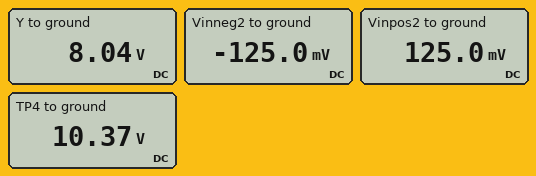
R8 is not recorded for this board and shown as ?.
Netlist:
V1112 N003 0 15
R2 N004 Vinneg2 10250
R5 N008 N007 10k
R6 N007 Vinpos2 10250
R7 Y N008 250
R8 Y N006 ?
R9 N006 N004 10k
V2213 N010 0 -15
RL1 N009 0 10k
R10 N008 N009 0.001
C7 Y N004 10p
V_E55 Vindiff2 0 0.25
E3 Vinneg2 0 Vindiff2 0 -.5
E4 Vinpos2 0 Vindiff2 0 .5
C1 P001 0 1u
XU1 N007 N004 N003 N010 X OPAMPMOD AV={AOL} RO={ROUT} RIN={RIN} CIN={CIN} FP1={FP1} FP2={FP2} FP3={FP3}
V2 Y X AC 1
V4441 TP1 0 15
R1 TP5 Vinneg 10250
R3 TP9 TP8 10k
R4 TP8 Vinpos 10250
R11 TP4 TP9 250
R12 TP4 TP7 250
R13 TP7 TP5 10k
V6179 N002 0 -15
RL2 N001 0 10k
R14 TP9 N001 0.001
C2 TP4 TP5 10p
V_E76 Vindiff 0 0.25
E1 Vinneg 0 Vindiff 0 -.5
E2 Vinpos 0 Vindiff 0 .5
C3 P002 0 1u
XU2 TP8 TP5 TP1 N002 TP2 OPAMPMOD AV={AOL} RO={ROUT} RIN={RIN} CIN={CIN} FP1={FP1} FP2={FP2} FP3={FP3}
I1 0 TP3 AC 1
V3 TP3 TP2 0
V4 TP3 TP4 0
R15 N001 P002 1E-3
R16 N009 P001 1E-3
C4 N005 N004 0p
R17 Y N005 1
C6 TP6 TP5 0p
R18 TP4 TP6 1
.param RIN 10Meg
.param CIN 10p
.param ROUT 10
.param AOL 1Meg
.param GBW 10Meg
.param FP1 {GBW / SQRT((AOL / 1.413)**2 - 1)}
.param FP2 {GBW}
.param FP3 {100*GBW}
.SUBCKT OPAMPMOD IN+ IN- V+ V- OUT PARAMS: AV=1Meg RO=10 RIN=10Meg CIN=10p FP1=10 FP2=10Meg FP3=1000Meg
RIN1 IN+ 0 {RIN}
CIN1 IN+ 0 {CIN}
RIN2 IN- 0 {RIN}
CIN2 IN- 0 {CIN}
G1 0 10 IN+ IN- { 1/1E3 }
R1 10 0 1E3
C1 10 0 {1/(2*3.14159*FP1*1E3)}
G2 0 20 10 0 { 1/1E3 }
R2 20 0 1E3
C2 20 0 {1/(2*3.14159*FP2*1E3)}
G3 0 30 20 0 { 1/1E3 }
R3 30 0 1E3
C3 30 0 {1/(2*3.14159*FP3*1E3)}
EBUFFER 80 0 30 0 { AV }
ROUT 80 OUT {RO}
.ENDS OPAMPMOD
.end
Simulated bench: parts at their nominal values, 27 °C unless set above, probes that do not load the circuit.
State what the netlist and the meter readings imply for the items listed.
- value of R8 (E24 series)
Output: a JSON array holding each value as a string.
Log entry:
["110 Ω"]
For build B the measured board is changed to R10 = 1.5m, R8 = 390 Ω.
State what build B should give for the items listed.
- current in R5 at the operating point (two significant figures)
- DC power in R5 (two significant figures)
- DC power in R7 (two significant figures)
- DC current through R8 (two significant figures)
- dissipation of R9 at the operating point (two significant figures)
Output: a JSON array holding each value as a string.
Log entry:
["680 µA", "4.7 mW", "1.1 mW", "710 µA", "5.0 mW"]
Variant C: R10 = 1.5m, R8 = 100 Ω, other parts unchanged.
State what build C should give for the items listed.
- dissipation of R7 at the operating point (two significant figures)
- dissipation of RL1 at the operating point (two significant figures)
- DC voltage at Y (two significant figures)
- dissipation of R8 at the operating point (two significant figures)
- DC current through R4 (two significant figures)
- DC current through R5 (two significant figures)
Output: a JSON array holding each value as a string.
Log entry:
["320 µW", "5.8 mW", "7.9 V", "16 µW", "490 µA", "370 µA"]
